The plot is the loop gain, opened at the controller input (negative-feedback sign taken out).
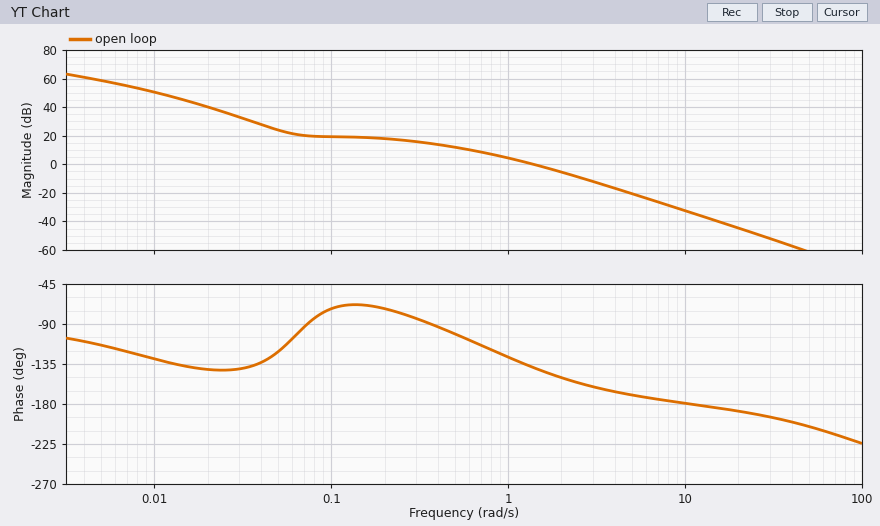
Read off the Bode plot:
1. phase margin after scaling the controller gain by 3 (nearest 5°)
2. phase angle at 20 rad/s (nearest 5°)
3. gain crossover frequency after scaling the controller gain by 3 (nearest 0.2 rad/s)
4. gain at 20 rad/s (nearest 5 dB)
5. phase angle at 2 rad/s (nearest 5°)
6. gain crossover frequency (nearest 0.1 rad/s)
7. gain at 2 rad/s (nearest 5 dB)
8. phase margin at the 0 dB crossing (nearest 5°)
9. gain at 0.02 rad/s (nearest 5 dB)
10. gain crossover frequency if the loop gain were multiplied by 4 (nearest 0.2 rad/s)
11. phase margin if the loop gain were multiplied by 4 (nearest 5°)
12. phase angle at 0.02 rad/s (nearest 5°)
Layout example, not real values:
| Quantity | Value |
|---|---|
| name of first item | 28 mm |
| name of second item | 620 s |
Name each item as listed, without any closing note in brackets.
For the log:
| Quantity | Value |
|---|---|
| phase margin after scaling the controller gain by 3 | 25° |
| phase angle at 20 rad/s | -190° |
| gain crossover frequency after scaling the controller gain by 3 | 2.6 rad/s |
| gain at 20 rad/s | -45 dB |
| phase angle at 2 rad/s | -150° |
| gain crossover frequency | 1.4 rad/s |
| gain at 2 rad/s | -5 dB |
| phase margin at the 0 dB crossing | 40° |
| gain at 0.02 rad/s | 40 dB |
| gain crossover frequency if the loop gain were multiplied by 4 | 3.0 rad/s |
| phase margin if the loop gain were multiplied by 4 | 20° |
| phase angle at 0.02 rad/s | -140° |
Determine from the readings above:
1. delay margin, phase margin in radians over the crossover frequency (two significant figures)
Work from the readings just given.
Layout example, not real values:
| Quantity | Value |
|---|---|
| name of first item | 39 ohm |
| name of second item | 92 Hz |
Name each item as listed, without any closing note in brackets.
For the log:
| Quantity | Value |
|---|---|
| delay margin, phase margin in radians over the crossover frequency | 0.50 s |
